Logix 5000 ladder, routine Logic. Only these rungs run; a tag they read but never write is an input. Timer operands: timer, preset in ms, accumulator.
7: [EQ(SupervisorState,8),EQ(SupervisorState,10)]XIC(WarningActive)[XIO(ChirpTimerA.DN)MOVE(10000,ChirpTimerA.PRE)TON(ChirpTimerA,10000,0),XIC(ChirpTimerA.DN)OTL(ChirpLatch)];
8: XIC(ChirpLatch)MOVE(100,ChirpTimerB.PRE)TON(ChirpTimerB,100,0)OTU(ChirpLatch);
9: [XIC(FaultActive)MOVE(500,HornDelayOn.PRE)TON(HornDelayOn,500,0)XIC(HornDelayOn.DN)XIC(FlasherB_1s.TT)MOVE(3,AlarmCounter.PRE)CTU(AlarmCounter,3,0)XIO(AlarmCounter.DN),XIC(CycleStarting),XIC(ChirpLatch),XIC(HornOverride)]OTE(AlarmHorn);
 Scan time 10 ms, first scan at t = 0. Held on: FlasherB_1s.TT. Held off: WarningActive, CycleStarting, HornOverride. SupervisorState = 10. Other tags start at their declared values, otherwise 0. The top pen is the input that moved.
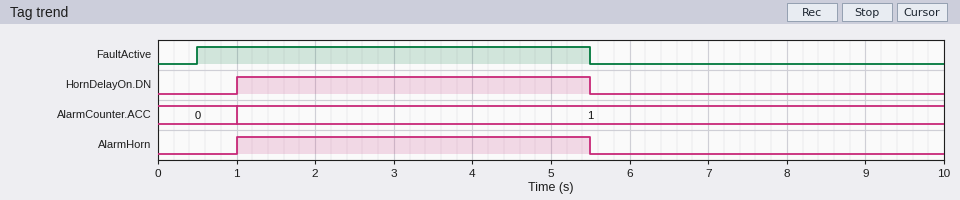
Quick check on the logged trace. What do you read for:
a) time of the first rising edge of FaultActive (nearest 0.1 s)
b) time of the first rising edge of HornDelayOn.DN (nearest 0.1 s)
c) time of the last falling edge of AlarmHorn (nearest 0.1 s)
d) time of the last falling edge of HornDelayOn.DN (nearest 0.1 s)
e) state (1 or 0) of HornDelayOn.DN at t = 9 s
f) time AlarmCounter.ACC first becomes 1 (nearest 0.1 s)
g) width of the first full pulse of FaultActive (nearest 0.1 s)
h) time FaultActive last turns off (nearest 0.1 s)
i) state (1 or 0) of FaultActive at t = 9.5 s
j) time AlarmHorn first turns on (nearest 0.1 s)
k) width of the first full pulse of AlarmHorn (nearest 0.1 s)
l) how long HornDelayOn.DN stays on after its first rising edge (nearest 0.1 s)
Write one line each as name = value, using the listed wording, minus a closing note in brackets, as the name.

time of the first rising edge of FaultActive = 0.5 s
time of the first rising edge of HornDelayOn.DN = 1.0 s
time of the last falling edge of AlarmHorn = 5.5 s
time of the last falling edge of HornDelayOn.DN = 5.5 s
state (1 or 0) of HornDelayOn.DN at t = 9 s = 0
time AlarmCounter.ACC first becomes 1 = 1.0 s
width of the first full pulse of FaultActive = 5.0 s
time FaultActive last turns off = 5.5 s
state (1 or 0) of FaultActive at t = 9.5 s = 0
time AlarmHorn first turns on = 1.0 s
width of the first full pulse of AlarmHorn = 4.5 s
how long HornDelayOn.DN stays on after its first rising edge = 4.5 s
